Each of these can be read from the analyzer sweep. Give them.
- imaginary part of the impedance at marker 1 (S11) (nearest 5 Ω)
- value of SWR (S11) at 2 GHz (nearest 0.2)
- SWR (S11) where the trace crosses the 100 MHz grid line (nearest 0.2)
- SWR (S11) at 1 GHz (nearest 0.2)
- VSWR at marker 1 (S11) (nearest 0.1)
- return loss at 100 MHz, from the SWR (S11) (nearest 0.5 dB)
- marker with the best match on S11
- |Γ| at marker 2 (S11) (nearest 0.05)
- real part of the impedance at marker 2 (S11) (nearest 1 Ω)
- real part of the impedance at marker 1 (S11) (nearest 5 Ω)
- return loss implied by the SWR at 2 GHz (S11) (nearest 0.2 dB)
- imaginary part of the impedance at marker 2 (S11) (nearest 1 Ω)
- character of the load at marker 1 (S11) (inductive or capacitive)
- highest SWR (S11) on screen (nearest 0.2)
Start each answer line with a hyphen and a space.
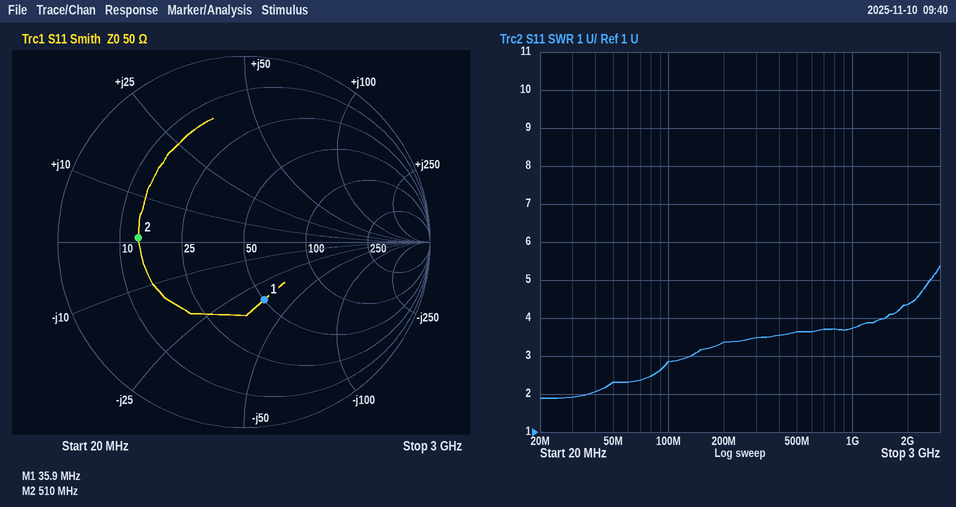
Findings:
- -35 Ω
- 4.4
- 2.8
- 3.8
- 2.0
- 6.5 dB
- marker 1
- 0.55
- 14 Ω
- 50 Ω
- 4.0 dB
- +1 Ω
- capacitive
- 5.4
